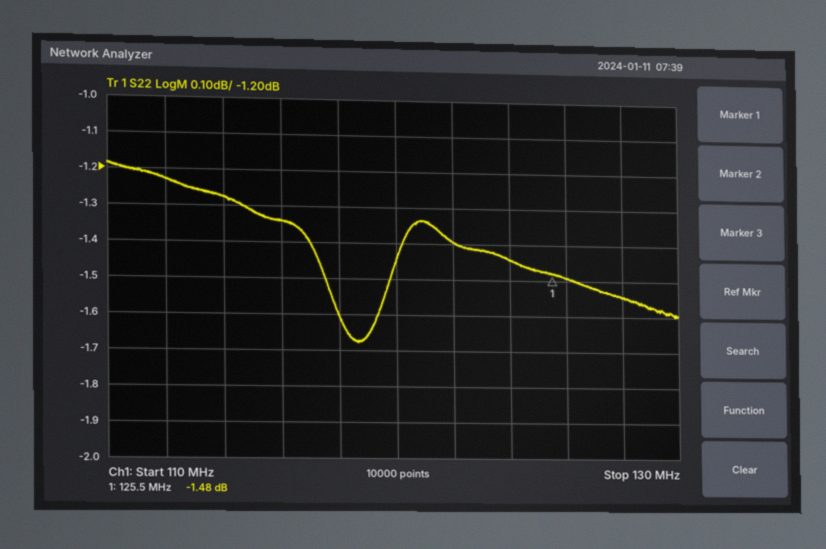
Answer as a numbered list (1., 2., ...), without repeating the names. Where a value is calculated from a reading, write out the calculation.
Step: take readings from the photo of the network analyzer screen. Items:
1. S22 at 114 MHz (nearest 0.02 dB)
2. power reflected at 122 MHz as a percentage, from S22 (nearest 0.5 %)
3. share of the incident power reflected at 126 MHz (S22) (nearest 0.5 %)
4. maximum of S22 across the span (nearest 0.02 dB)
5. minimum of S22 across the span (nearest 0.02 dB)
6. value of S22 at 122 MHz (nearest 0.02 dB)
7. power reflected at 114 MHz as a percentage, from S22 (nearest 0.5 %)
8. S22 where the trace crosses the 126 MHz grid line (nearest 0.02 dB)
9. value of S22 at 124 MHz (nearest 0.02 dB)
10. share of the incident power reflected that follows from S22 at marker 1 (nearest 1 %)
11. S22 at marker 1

1. -1.28 dB
2. 10^(-1.4/10) ≈ 72.4 %, so 72.5 % to the nearest 0.5 %
3. 10^(-1.5/10) ≈ 70.8 %, so 71.0 % to the nearest 0.5 %
4. -1.18 dB
5. -1.68 dB
6. -1.40 dB
7. 10^(-1.28/10) ≈ 74.5 %
8. -1.50 dB
9. -1.44 dB
10. 10^(-1.48/10) ≈ 71 %
11. -1.48 dB
